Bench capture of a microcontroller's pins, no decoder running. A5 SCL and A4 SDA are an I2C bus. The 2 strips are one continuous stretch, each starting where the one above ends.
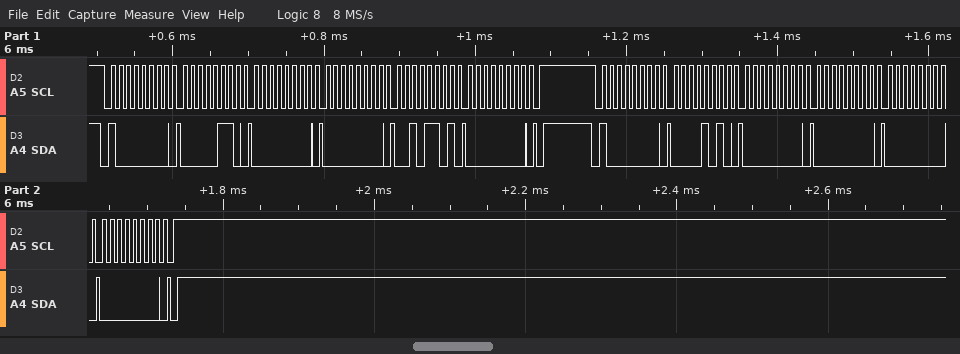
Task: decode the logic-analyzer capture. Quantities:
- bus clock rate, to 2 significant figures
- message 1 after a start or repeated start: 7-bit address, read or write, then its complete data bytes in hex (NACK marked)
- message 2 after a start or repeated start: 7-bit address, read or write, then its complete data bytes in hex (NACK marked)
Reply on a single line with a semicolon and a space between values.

100 kHz; 0x40 write: 06 00 00 2D 00; 0x40 write: 0A 00 00 00 00
